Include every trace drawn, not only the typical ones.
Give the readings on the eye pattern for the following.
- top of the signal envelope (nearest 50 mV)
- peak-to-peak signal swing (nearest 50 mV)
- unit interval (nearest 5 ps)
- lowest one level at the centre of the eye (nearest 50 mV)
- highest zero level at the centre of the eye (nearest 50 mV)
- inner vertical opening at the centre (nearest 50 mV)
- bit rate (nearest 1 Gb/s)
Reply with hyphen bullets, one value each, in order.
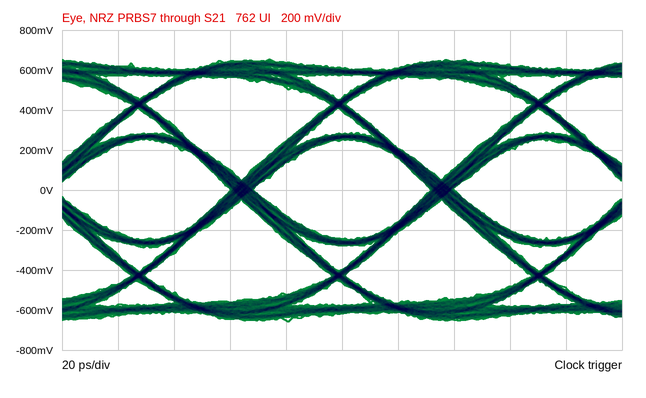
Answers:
- 650 mV
- 1.30 V
- 70 ps
- 250 mV
- -250 mV
- 500 mV
- 14 Gb/s
